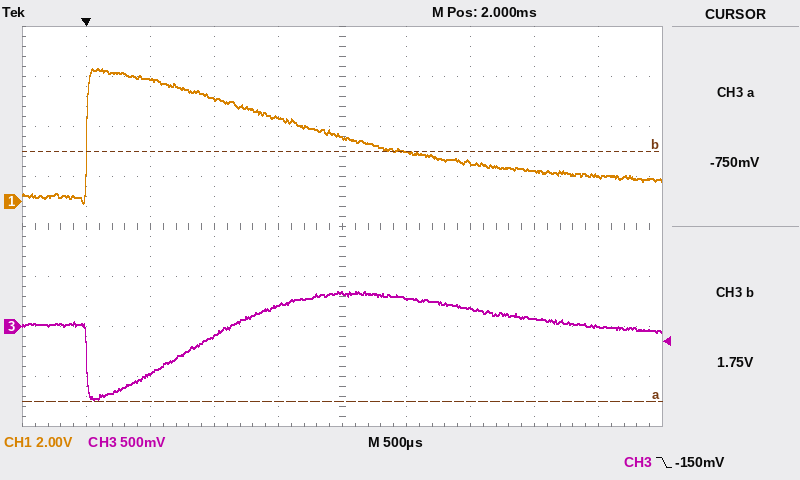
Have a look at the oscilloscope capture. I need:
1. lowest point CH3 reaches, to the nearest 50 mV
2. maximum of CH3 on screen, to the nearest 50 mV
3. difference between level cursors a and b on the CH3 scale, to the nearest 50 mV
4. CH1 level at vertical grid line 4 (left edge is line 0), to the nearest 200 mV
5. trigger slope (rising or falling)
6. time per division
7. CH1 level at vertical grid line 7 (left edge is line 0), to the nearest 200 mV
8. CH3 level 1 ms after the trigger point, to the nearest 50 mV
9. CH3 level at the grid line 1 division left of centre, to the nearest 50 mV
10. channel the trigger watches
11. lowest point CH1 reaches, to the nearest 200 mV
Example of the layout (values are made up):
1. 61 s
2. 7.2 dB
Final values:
1. -750 mV
2. 350 mV
3. 2.50 V
4. 3.4 V
5. falling
6. 500 µs
7. 1.6 V
8. -100 mV
9. 200 mV
10. CH3
11. 0.0 V
